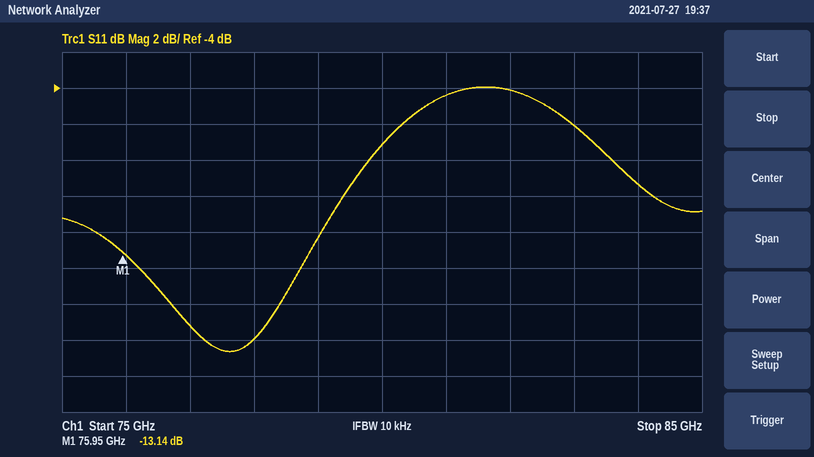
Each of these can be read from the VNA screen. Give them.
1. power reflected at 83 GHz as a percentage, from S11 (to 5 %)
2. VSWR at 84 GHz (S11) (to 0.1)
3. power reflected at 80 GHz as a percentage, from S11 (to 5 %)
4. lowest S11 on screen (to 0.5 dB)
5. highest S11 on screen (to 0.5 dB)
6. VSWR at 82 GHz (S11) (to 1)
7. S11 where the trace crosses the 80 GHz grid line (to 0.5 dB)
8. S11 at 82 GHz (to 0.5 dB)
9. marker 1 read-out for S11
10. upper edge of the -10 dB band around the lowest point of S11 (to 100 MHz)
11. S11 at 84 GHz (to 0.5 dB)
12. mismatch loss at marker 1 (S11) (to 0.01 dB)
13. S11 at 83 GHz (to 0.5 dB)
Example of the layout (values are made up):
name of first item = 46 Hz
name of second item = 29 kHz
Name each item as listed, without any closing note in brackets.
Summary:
power reflected at 83 GHz as a percentage, from S11 = 25 %
VSWR at 84 GHz (S11) = 2.0
power reflected at 80 GHz as a percentage, from S11 = 20 %
lowest S11 on screen = -18.5 dB
highest S11 on screen = -4.0 dB
VSWR at 82 GHz (S11) = 4
S11 where the trace crosses the 80 GHz grid line = -7.0 dB
S11 at 82 GHz = -4.0 dB
marker 1 read-out for S11 = -13.14 dB
upper edge of the -10 dB band around the lowest point of S11 = 79.4 GHz
S11 at 84 GHz = -9.5 dB
mismatch loss at marker 1 (S11) = 0.22 dB
S11 at 83 GHz = -6.0 dB
